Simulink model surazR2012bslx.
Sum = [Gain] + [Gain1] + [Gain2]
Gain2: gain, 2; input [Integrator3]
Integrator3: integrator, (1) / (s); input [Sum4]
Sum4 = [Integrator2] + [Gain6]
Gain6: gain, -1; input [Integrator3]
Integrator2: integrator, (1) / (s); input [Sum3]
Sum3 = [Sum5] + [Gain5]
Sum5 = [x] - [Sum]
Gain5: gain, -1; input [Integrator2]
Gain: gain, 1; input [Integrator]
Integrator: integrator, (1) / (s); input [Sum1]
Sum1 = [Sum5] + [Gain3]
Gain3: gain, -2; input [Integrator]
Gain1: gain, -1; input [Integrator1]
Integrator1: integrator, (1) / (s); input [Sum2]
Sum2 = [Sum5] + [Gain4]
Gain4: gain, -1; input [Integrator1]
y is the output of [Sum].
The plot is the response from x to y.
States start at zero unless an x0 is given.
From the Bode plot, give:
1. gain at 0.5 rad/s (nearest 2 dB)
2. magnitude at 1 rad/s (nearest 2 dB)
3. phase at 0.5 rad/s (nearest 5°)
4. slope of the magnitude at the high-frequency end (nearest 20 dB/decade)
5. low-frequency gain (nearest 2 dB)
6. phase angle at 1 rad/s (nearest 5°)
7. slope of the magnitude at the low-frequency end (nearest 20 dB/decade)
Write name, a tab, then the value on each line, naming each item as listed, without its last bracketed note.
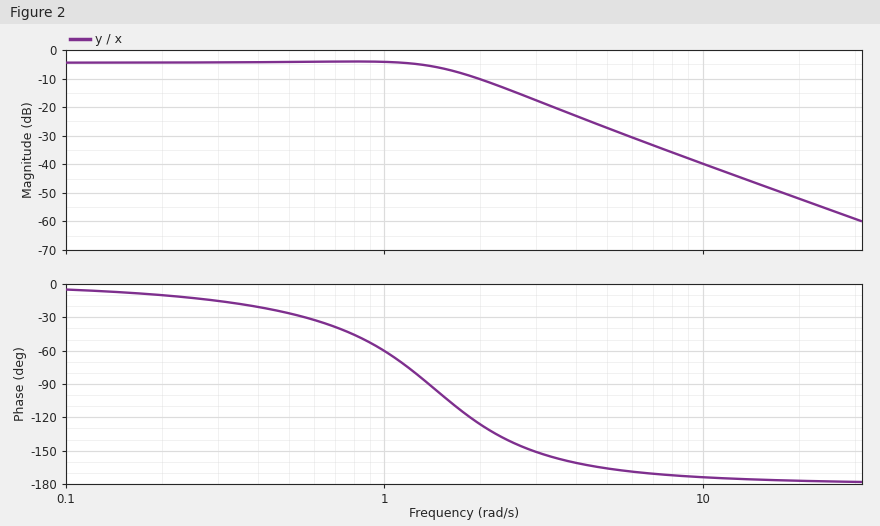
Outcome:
gain at 0.5 rad/s	-4 dB
magnitude at 1 rad/s	-4 dB
phase at 0.5 rad/s	-25°
slope of the magnitude at the high-frequency end	-40 dB/decade
low-frequency gain	-4 dB
phase angle at 1 rad/s	-60°
slope of the magnitude at the low-frequency end	0 dB/decade
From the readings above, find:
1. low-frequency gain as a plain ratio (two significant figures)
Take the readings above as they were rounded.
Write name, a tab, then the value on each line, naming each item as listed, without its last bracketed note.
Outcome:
low-frequency gain as a plain ratio	0.63
